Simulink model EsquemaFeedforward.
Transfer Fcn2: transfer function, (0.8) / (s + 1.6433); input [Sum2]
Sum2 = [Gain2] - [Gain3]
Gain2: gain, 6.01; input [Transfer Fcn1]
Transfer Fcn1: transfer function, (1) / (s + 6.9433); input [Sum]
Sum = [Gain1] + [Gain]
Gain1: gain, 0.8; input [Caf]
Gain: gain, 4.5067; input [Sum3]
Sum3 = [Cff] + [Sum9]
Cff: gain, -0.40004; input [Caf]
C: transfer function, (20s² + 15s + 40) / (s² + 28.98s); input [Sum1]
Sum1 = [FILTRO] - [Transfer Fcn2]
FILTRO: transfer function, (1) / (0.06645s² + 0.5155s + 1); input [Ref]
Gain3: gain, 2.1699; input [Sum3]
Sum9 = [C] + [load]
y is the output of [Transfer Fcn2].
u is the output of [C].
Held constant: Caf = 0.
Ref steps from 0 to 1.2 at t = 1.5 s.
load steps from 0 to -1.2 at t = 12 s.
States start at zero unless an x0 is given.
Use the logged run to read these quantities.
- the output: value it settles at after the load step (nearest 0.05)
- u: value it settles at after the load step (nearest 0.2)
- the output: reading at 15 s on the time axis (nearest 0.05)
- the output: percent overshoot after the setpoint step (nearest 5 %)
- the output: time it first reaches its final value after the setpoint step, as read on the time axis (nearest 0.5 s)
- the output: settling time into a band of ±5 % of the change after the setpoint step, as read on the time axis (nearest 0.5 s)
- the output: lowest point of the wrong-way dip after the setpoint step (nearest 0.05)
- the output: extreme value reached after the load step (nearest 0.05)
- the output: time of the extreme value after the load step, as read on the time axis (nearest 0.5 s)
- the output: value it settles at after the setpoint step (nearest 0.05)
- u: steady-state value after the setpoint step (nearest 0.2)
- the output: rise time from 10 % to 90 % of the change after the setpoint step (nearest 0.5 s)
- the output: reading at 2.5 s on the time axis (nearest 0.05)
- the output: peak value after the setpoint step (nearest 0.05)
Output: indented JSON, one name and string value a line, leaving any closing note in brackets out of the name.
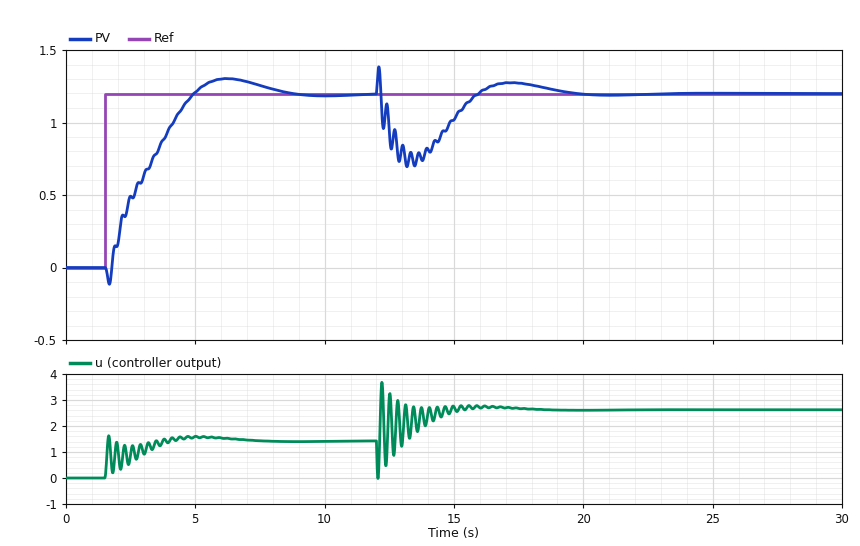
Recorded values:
{
  "the output: value it settles at after the load step": "1.20",
  "u: value it settles at after the load step": "2.6",
  "the output: reading at 15 s on the time axis": "1.00",
  "the output: percent overshoot after the setpoint step": "10 %",
  "the output: time it first reaches its final value after the setpoint step, as read on the time axis": "5.0 s",
  "the output: settling time into a band of ±5 % of the change after the setpoint step, as read on the time axis": "7.5 s",
  "the output: lowest point of the wrong-way dip after the setpoint step": "-0.10",
  "the output: extreme value reached after the load step": "0.70",
  "the output: time of the extreme value after the load step, as read on the time axis": "13.0 s",
  "the output: value it settles at after the setpoint step": "1.20",
  "u: steady-state value after the setpoint step": "1.4",
  "the output: rise time from 10 % to 90 % of the change after the setpoint step": "2.5 s",
  "the output: reading at 2.5 s on the time axis": "0.50",
  "the output: peak value after the setpoint step": "1.30"
}
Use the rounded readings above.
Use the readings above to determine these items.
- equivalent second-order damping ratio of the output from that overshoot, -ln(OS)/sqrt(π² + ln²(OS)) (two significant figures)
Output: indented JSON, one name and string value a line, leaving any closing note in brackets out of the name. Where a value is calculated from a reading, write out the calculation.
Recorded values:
{
  "equivalent second-order damping ratio of the output from that overshoot, -ln(OS)/sqrt(π² + ln²(OS))": "ln(0.1) = -2.303; 2.303 / sqrt(9.870 + 5.302) = 0.59"
}
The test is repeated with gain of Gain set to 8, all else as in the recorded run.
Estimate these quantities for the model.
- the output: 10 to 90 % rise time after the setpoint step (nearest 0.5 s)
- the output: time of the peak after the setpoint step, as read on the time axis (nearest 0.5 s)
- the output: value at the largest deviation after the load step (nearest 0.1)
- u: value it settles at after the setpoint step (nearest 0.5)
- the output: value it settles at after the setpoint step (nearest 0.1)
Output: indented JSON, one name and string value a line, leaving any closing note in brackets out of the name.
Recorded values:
{
  "the output: 10 to 90 % rise time after the setpoint step": "2.0 s",
  "the output: time of the peak after the setpoint step, as read on the time axis": "5.0 s",
  "the output: value at the largest deviation after the load step": "0.5",
  "u: value it settles at after the setpoint step": "0.5",
  "the output: value it settles at after the setpoint step": "1.2"
}
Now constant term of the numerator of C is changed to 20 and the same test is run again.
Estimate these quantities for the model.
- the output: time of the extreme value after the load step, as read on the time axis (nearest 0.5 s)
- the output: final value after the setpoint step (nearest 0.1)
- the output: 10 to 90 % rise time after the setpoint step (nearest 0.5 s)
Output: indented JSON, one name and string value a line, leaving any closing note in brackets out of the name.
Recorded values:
{
  "the output: time of the extreme value after the load step, as read on the time axis": "13.5 s",
  "the output: final value after the setpoint step": "1.2",
  "the output: 10 to 90 % rise time after the setpoint step": "4.5 s"
}
